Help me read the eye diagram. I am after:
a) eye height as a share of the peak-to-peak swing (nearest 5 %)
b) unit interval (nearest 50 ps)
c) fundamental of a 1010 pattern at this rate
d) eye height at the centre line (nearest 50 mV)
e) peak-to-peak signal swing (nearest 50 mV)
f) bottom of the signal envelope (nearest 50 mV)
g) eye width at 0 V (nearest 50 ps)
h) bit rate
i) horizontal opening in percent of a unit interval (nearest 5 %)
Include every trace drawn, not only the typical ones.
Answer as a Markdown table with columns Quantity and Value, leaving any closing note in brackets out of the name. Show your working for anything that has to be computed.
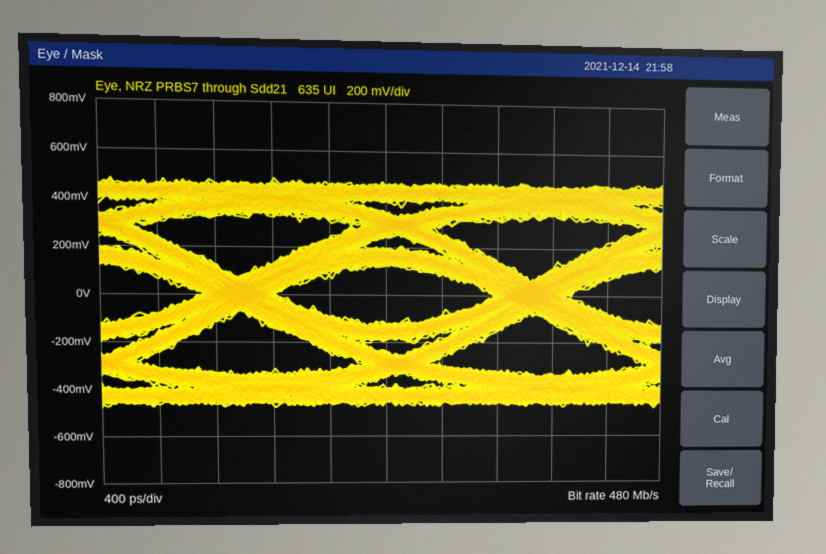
| Quantity | Value |
|---|---|
| eye height as a share of the peak-to-peak swing | 250 mV / 950 mV ≈ 26.3 %, so 25 % to the nearest 5 % |
| unit interval | 2.10 ns |
| fundamental of a 1010 pattern at this rate | 240 MHz |
| eye height at the centre line | 250 mV |
| peak-to-peak signal swing | 950 mV |
| bottom of the signal envelope | -500 mV |
| eye width at 0 V | 1.55 ns |
| bit rate | 480 Mb/s |
| horizontal opening in percent of a unit interval | 1.55 ns / 2.10 ns ≈ 73.8 %, so 75 % to the nearest 5 % |
